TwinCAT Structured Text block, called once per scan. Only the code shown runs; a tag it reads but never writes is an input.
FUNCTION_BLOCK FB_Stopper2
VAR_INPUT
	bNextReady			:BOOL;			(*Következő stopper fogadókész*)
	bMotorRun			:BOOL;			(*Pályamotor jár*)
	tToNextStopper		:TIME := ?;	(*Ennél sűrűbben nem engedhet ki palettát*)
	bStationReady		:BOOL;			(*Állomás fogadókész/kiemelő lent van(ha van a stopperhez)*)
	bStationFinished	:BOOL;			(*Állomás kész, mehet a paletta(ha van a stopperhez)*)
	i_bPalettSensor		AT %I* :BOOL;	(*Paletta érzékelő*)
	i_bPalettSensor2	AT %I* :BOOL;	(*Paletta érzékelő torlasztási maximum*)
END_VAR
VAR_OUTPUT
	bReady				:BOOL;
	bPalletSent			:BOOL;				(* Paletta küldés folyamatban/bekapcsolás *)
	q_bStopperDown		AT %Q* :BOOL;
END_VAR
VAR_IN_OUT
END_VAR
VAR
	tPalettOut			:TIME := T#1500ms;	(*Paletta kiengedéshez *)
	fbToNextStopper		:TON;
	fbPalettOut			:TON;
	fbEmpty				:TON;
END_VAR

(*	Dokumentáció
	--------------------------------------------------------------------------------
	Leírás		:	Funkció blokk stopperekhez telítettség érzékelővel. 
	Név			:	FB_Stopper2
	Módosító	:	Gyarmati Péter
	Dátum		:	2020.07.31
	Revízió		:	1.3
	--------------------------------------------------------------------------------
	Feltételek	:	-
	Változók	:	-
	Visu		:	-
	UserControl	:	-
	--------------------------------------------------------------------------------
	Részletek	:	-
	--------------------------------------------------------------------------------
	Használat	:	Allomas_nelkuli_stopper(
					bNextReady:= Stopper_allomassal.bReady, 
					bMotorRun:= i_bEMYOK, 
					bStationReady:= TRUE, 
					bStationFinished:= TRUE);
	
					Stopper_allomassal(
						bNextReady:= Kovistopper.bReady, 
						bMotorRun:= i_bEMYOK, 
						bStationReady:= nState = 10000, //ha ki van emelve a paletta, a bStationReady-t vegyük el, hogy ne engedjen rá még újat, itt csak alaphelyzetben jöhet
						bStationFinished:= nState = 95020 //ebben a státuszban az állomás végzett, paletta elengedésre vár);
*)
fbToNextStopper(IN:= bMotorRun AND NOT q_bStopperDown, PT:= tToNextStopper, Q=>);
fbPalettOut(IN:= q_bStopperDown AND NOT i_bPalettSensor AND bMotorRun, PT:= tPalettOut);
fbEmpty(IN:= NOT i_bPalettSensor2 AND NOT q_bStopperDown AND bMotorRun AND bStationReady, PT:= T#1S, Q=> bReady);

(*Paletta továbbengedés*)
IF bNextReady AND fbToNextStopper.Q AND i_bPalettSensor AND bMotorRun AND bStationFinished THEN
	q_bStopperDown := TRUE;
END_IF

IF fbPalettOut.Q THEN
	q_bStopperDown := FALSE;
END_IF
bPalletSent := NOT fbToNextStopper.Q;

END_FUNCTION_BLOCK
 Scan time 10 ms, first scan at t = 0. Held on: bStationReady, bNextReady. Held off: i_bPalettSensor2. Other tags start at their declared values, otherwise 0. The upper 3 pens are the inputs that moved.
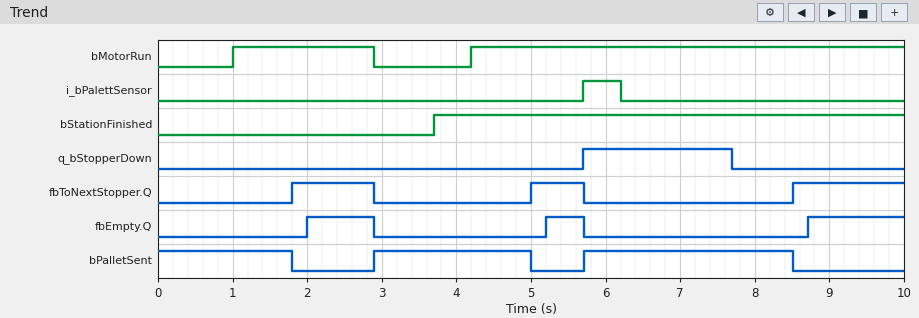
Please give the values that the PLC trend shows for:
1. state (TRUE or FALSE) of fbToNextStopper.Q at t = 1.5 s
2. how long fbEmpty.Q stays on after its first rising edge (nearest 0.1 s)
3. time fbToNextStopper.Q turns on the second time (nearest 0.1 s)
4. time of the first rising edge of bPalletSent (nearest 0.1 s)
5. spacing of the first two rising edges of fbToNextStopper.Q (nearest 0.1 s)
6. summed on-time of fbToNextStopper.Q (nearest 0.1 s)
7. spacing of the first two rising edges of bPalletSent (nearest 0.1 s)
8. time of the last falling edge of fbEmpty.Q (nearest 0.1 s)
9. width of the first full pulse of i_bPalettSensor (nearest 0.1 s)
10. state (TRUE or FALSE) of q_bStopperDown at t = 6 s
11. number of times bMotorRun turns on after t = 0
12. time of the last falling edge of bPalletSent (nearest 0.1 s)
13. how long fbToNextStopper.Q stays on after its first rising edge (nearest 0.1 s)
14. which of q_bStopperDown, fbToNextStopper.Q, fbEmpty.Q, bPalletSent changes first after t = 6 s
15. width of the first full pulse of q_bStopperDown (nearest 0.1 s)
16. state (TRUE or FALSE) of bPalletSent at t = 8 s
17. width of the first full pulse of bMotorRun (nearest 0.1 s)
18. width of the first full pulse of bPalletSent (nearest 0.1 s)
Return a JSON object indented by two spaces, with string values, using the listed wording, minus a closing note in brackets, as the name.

{
  "state (TRUE or FALSE) of fbToNextStopper.Q at t = 1.5 s": "FALSE",
  "how long fbEmpty.Q stays on after its first rising edge": "0.9 s",
  "time fbToNextStopper.Q turns on the second time": "5.0 s",
  "time of the first rising edge of bPalletSent": "2.9 s",
  "spacing of the first two rising edges of fbToNextStopper.Q": "3.2 s",
  "summed on-time of fbToNextStopper.Q": "3.3 s",
  "spacing of the first two rising edges of bPalletSent": "2.8 s",
  "time of the last falling edge of fbEmpty.Q": "5.7 s",
  "width of the first full pulse of i_bPalettSensor": "0.5 s",
  "state (TRUE or FALSE) of q_bStopperDown at t = 6 s": "TRUE",
  "number of times bMotorRun turns on after t = 0": "2",
  "time of the last falling edge of bPalletSent": "8.5 s",
  "how long fbToNextStopper.Q stays on after its first rising edge": "1.1 s",
  "which of q_bStopperDown, fbToNextStopper.Q, fbEmpty.Q, bPalletSent changes first after t = 6 s": "q_bStopperDown",
  "width of the first full pulse of q_bStopperDown": "2.0 s",
  "state (TRUE or FALSE) of bPalletSent at t = 8 s": "TRUE",
  "width of the first full pulse of bMotorRun": "1.9 s",
  "width of the first full pulse of bPalletSent": "2.1 s"
}
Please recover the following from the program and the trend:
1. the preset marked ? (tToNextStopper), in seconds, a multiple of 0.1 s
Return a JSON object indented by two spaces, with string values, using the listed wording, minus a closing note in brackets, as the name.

{
  "the preset marked ? (tToNextStopper), in seconds, a multiple of 0.1 s": "0.8 s"
}
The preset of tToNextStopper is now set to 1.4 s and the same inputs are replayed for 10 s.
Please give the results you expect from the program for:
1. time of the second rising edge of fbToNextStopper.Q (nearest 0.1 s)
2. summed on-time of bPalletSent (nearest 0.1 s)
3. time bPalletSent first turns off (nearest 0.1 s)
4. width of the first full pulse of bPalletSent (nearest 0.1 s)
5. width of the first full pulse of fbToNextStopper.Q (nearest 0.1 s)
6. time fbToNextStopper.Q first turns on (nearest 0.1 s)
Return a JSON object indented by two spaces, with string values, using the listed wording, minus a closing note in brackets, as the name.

{
  "time of the second rising edge of fbToNextStopper.Q": "5.6 s",
  "summed on-time of bPalletSent": "8.5 s",
  "time bPalletSent first turns off": "2.4 s",
  "width of the first full pulse of bPalletSent": "2.7 s",
  "width of the first full pulse of fbToNextStopper.Q": "0.5 s",
  "time fbToNextStopper.Q first turns on": "2.4 s"
}
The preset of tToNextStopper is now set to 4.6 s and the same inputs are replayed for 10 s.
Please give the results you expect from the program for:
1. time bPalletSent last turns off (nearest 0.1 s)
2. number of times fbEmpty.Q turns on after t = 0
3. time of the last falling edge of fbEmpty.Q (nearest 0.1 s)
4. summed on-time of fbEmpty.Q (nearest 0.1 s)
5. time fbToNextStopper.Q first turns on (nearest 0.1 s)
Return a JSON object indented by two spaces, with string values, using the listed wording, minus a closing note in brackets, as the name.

{
  "time bPalletSent last turns off": "8.8 s",
  "number of times fbEmpty.Q turns on after t = 0": "2",
  "time of the last falling edge of fbEmpty.Q": "2.9 s",
  "summed on-time of fbEmpty.Q": "5.7 s",
  "time fbToNextStopper.Q first turns on": "8.8 s"
}
